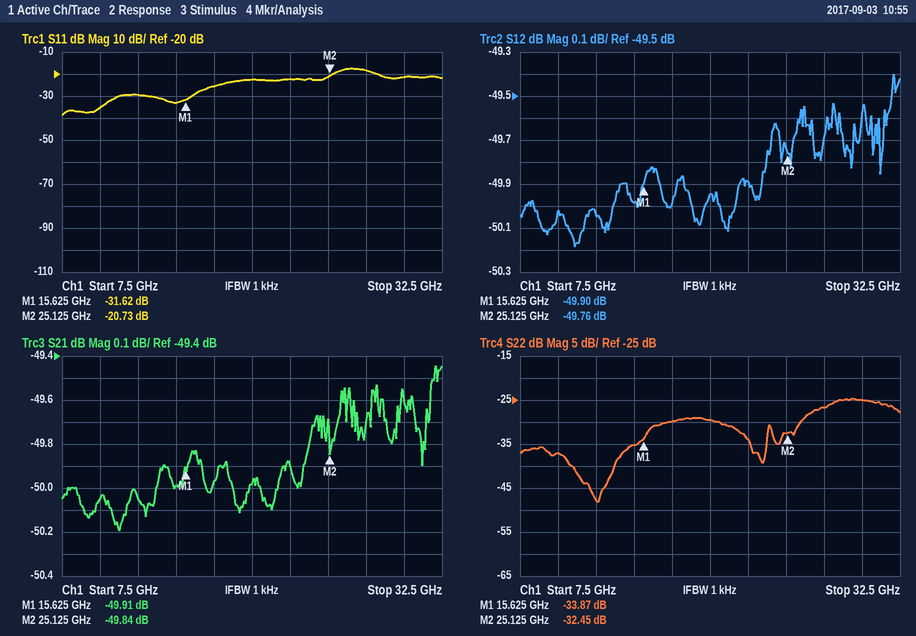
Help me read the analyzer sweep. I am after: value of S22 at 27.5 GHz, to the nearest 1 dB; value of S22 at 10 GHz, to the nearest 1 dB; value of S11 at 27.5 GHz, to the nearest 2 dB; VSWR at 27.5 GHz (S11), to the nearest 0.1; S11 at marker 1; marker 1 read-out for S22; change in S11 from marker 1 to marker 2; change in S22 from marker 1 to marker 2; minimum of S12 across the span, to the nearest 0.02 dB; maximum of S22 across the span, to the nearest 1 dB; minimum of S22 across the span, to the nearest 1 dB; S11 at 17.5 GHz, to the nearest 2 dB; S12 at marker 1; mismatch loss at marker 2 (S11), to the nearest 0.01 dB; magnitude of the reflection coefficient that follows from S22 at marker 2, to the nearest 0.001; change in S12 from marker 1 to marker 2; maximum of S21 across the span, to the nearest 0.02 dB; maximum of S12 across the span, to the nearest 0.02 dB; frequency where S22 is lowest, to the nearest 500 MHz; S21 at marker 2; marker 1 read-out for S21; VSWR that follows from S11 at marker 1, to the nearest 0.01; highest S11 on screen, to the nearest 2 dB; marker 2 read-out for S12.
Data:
-27 dB
-37 dB
-18 dB
1.3
-31.62 dB
-33.87 dB
10.89 dB
1.42 dB
-50.18 dB
-25 dB
-48 dB
-26 dB
-49.90 dB
0.04 dB
0.024
0.14 dB
-49.44 dB
-49.40 dB
12.5 GHz
-49.84 dB
-49.91 dB
1.05
-18 dB
-49.76 dB
